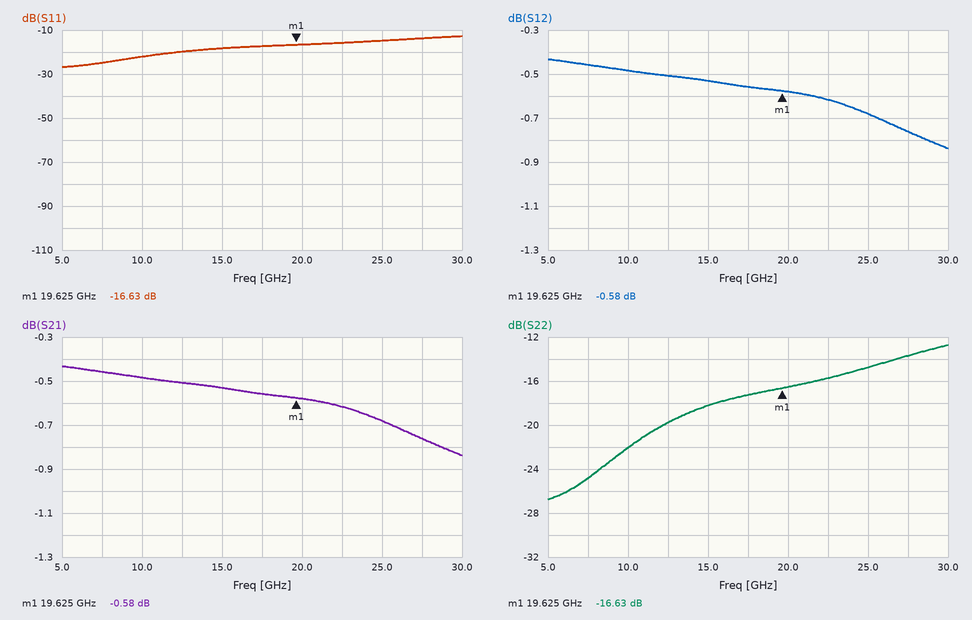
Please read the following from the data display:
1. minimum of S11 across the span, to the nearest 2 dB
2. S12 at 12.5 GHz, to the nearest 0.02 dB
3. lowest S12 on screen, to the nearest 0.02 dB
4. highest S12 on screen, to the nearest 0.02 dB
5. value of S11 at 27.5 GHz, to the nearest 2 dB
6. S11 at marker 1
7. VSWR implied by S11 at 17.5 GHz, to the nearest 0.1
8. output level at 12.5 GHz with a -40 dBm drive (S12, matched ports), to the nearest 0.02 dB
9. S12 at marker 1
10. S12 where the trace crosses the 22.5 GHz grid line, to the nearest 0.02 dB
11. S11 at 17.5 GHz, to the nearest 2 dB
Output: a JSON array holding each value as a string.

["-26 dB", "-0.50 dB", "-0.84 dB", "-0.44 dB", "-14 dB", "-16.63 dB", "1.3", "-40.50 dBm", "-0.58 dB", "-0.62 dB", "-18 dB"]
